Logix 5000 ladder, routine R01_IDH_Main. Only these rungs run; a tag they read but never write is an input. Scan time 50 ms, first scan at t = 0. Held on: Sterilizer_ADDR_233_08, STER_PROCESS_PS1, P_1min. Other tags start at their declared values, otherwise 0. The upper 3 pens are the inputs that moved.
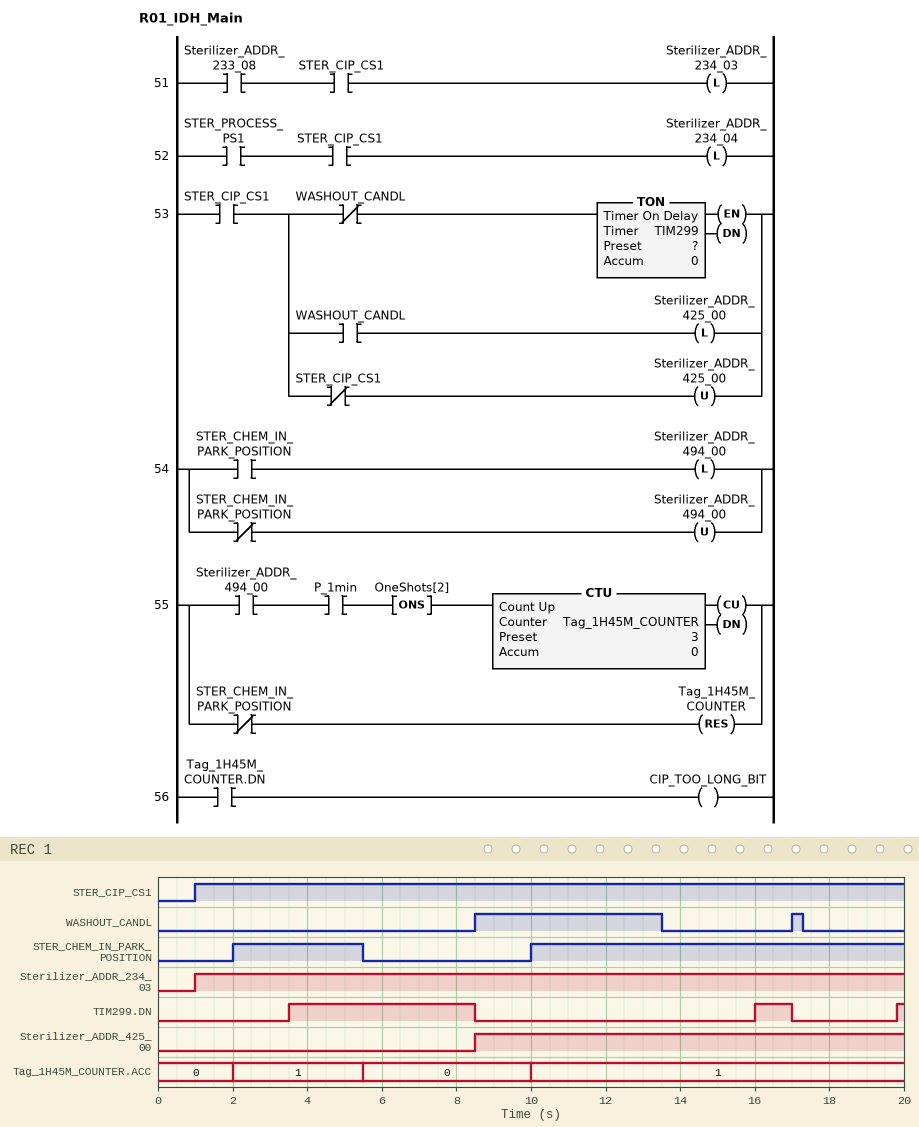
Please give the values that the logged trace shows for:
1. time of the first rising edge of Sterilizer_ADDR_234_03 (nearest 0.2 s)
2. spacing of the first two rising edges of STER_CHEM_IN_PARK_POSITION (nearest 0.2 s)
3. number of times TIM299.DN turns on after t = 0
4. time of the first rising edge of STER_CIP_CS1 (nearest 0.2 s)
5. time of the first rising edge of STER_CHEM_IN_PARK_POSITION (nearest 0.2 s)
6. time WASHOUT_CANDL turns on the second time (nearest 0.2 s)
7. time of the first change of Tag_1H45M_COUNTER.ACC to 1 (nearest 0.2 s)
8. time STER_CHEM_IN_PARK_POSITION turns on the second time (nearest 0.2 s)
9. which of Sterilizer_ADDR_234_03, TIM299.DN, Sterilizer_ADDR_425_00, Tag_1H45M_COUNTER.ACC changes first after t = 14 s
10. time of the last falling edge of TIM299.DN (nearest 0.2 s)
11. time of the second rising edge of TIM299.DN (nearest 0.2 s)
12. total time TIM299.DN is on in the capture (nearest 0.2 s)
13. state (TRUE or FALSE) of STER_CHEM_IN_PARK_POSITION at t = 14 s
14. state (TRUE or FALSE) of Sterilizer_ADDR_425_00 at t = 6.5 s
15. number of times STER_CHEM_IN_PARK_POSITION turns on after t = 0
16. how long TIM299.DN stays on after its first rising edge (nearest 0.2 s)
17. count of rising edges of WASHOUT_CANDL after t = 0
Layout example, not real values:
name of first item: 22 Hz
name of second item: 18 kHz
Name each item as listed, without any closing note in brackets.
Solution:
time of the first rising edge of Sterilizer_ADDR_234_03: 1.0 s
spacing of the first two rising edges of STER_CHEM_IN_PARK_POSITION: 8.0 s
number of times TIM299.DN turns on after t = 0: 3
time of the first rising edge of STER_CIP_CS1: 1.0 s
time of the first rising edge of STER_CHEM_IN_PARK_POSITION: 2.0 s
time WASHOUT_CANDL turns on the second time: 17.0 s
time of the first change of Tag_1H45M_COUNTER.ACC to 1: 2.0 s
time STER_CHEM_IN_PARK_POSITION turns on the second time: 10.0 s
which of Sterilizer_ADDR_234_03, TIM299.DN, Sterilizer_ADDR_425_00, Tag_1H45M_COUNTER.ACC changes first after t = 14 s: TIM299.DN
time of the last falling edge of TIM299.DN: 17.0 s
time of the second rising edge of TIM299.DN: 16.0 s
total time TIM299.DN is on in the capture: 6.2 s
state (TRUE or FALSE) of STER_CHEM_IN_PARK_POSITION at t = 14 s: TRUE
state (TRUE or FALSE) of Sterilizer_ADDR_425_00 at t = 6.5 s: FALSE
number of times STER_CHEM_IN_PARK_POSITION turns on after t = 0: 2
how long TIM299.DN stays on after its first rising edge: 5.0 s
count of rising edges of WASHOUT_CANDL after t = 0: 2
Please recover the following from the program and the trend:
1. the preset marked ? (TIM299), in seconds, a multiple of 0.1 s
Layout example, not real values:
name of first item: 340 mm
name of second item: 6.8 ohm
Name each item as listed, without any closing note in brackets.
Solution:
the preset marked ? (TIM299), in seconds, a multiple of 0.1 s: 2.5 s
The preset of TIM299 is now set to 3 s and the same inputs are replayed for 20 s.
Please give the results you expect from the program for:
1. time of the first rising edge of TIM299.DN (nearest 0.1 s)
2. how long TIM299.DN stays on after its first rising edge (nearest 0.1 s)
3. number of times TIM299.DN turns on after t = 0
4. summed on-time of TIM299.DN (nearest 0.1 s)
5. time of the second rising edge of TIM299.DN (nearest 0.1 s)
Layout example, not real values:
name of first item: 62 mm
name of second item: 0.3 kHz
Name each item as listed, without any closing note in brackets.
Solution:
time of the first rising edge of TIM299.DN: 4.0 s
how long TIM299.DN stays on after its first rising edge: 4.5 s
number of times TIM299.DN turns on after t = 0: 2
summed on-time of TIM299.DN: 5.0 s
time of the second rising edge of TIM299.DN: 16.5 s
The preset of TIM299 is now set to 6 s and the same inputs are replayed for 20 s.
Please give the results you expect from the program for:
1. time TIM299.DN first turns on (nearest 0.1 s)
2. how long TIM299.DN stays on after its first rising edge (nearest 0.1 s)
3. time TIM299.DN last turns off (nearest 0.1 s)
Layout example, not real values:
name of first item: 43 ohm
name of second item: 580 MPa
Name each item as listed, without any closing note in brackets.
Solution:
time TIM299.DN first turns on: 7.0 s
how long TIM299.DN stays on after its first rising edge: 1.5 s
time TIM299.DN last turns off: 8.5 s
